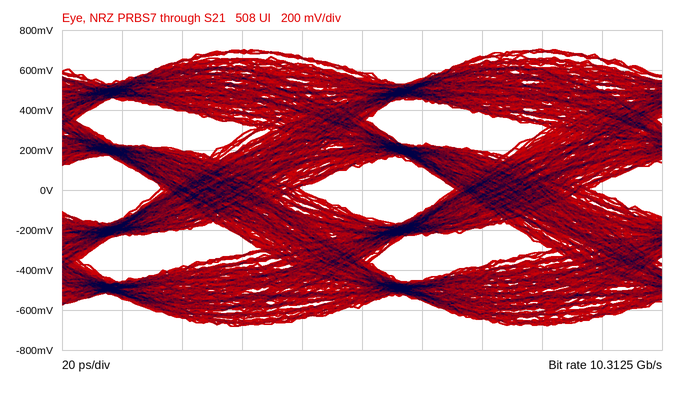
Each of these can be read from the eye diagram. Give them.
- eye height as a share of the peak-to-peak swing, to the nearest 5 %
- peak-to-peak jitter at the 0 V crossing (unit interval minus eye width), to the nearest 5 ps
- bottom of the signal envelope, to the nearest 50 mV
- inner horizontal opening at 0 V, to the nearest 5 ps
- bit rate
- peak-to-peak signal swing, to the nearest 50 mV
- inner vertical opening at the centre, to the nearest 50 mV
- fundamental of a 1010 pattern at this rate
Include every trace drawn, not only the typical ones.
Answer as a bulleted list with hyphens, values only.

- 20 %
- 45 ps
- -700 mV
- 50 ps
- 10.3125 Gb/s
- 1.40 V
- 250 mV
- 5.15625 GHz
